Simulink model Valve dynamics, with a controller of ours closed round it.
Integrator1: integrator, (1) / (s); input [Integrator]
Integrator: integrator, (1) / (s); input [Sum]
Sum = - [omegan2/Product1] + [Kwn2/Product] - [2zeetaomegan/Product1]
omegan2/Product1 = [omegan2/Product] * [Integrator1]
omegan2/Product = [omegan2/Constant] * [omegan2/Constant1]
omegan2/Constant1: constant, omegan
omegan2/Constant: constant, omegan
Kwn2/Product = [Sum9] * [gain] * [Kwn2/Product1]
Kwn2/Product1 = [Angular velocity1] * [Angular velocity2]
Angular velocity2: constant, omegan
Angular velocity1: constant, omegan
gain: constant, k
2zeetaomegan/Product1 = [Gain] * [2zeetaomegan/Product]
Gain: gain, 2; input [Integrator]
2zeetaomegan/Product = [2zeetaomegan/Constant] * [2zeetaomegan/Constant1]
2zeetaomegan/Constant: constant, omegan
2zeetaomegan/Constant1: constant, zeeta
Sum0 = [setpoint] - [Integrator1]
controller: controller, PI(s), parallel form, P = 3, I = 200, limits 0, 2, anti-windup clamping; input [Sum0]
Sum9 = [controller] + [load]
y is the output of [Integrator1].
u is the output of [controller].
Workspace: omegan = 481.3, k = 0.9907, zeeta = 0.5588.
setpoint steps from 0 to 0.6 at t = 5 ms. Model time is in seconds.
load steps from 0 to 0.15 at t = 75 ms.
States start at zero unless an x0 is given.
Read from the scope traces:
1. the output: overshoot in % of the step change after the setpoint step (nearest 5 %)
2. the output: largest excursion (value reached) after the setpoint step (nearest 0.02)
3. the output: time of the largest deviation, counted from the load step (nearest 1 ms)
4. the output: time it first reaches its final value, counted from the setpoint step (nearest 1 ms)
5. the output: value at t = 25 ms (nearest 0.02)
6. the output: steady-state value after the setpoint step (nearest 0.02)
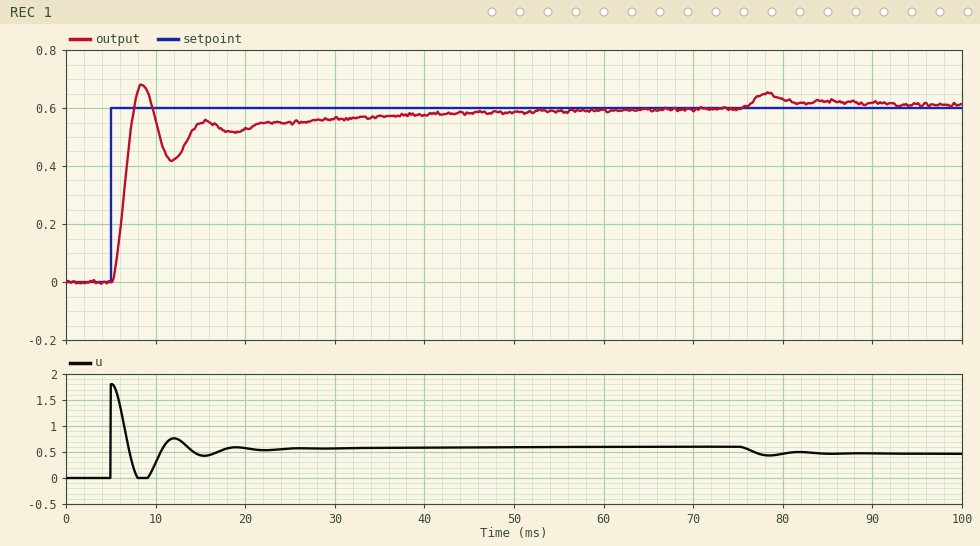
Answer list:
15 %
0.68
3 ms
3 ms
0.54
0.60
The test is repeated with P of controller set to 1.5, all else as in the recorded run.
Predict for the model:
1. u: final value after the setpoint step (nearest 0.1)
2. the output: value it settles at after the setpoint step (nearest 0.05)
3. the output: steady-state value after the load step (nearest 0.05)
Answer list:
0.6
0.60
0.60
